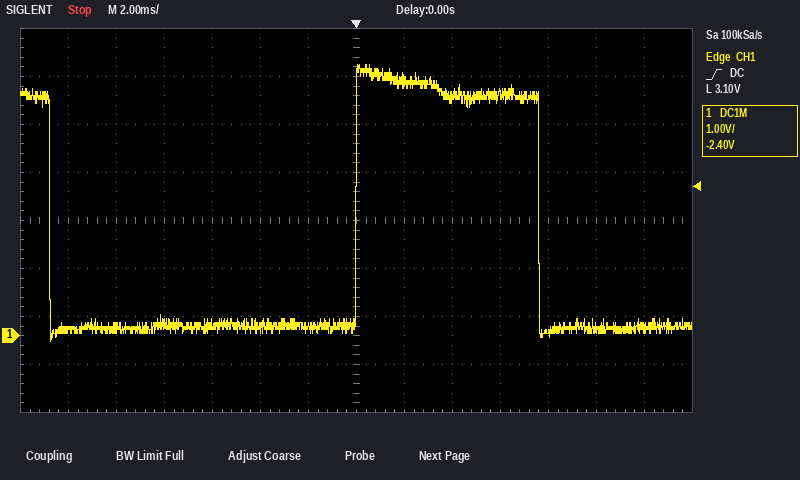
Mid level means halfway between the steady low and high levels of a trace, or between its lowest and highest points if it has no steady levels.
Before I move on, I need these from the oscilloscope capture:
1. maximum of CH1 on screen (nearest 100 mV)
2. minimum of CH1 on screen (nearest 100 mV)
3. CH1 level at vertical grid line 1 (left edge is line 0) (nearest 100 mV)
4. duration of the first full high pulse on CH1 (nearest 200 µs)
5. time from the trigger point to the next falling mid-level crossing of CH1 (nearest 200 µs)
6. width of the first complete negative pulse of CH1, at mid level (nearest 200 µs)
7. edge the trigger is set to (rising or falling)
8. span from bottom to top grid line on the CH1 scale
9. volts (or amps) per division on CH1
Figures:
5.6 V
-100 mV
100 mV
7.6 ms
7.6 ms
12.8 ms
rising
8 V
1 V
